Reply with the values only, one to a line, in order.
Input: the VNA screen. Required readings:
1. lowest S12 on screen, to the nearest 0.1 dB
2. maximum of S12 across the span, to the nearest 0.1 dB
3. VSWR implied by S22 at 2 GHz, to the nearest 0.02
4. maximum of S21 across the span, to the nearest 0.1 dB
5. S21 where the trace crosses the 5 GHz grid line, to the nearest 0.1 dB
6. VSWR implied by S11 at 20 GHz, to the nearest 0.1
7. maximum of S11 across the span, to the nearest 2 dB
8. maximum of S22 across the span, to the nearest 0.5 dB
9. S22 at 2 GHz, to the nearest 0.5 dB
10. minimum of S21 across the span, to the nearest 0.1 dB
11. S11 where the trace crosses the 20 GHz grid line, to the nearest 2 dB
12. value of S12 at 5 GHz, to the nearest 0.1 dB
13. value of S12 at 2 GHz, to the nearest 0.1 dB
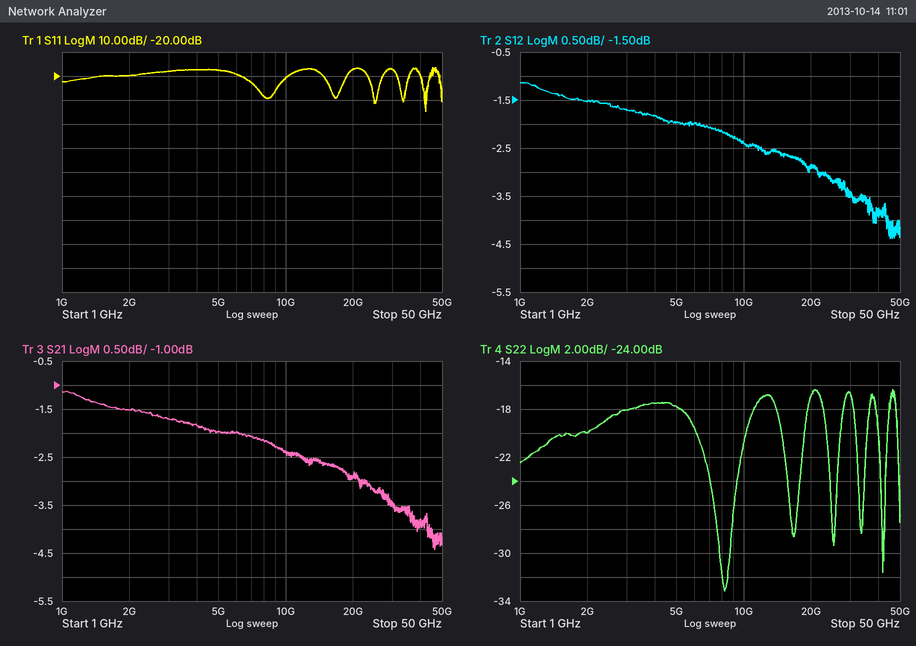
-4.4 dB
-1.1 dB
1.22
-1.1 dB
-2.0 dB
1.3
-16 dB
-16.5 dB
-20.0 dB
-4.4 dB
-18 dB
-2.0 dB
-1.5 dB
